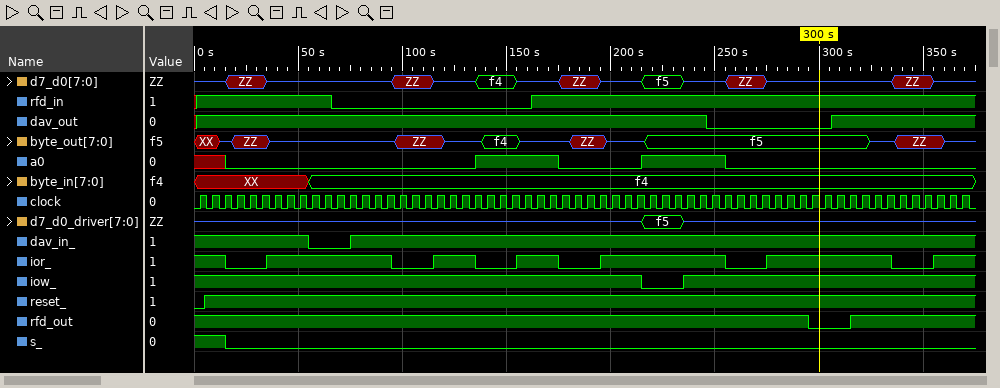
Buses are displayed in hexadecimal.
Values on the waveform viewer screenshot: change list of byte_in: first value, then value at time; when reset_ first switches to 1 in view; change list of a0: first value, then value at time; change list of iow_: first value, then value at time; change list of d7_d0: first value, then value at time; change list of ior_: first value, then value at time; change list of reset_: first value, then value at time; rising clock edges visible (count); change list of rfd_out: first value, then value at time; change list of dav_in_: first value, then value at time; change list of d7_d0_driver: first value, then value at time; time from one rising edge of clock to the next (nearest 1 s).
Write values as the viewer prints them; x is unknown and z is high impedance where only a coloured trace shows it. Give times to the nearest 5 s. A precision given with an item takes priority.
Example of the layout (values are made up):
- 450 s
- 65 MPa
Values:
- XX, f4 at 55 s
- 5 s
- x, 0 at 15 s, 1 at 135 s, 0 at 175 s, 1 at 215 s, 0 at 255 s
- 1, 0 at 215 s, 1 at 235 s
- z, ZZ at 15 s, z at 35 s, ZZ at 95 s, z at 115 s, f4 at 135 s, z at 155 s, ZZ at 175 s, z at 195 s, f5 at 215 s, z at 235 s, ZZ at 255 s, z at 275 s, ZZ at 335 s, z at 355 s
- 1, 0 at 15 s, 1 at 35 s, 0 at 95 s, 1 at 115 s, 0 at 135 s, 1 at 155 s, 0 at 175 s, 1 at 195 s, 0 at 255 s, 1 at 275 s, 0 at 335 s, 1 at 355 s
- 0, 1 at 5 s
- 62
- 1, 0 at 295 s, 1 at 315 s
- 1, 0 at 55 s, 1 at 75 s
- z, f5 at 215 s, z at 235 s
- 6 s
